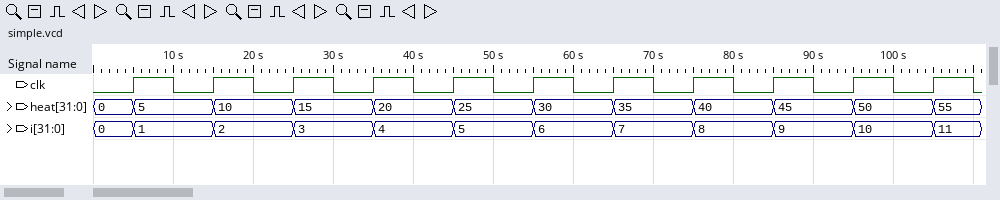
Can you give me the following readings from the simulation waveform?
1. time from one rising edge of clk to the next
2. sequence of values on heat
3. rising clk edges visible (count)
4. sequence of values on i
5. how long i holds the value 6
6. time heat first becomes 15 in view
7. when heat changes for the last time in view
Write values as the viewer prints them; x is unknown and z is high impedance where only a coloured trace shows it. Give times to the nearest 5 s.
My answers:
10 s
0, 5, 10, 15, 20, 25, 30, 35, 40, 45, 50, 55
11
0, 1, 2, 3, 4, 5, 6, 7, 8, 9, 10, 11
10 s
25 s
105 s
